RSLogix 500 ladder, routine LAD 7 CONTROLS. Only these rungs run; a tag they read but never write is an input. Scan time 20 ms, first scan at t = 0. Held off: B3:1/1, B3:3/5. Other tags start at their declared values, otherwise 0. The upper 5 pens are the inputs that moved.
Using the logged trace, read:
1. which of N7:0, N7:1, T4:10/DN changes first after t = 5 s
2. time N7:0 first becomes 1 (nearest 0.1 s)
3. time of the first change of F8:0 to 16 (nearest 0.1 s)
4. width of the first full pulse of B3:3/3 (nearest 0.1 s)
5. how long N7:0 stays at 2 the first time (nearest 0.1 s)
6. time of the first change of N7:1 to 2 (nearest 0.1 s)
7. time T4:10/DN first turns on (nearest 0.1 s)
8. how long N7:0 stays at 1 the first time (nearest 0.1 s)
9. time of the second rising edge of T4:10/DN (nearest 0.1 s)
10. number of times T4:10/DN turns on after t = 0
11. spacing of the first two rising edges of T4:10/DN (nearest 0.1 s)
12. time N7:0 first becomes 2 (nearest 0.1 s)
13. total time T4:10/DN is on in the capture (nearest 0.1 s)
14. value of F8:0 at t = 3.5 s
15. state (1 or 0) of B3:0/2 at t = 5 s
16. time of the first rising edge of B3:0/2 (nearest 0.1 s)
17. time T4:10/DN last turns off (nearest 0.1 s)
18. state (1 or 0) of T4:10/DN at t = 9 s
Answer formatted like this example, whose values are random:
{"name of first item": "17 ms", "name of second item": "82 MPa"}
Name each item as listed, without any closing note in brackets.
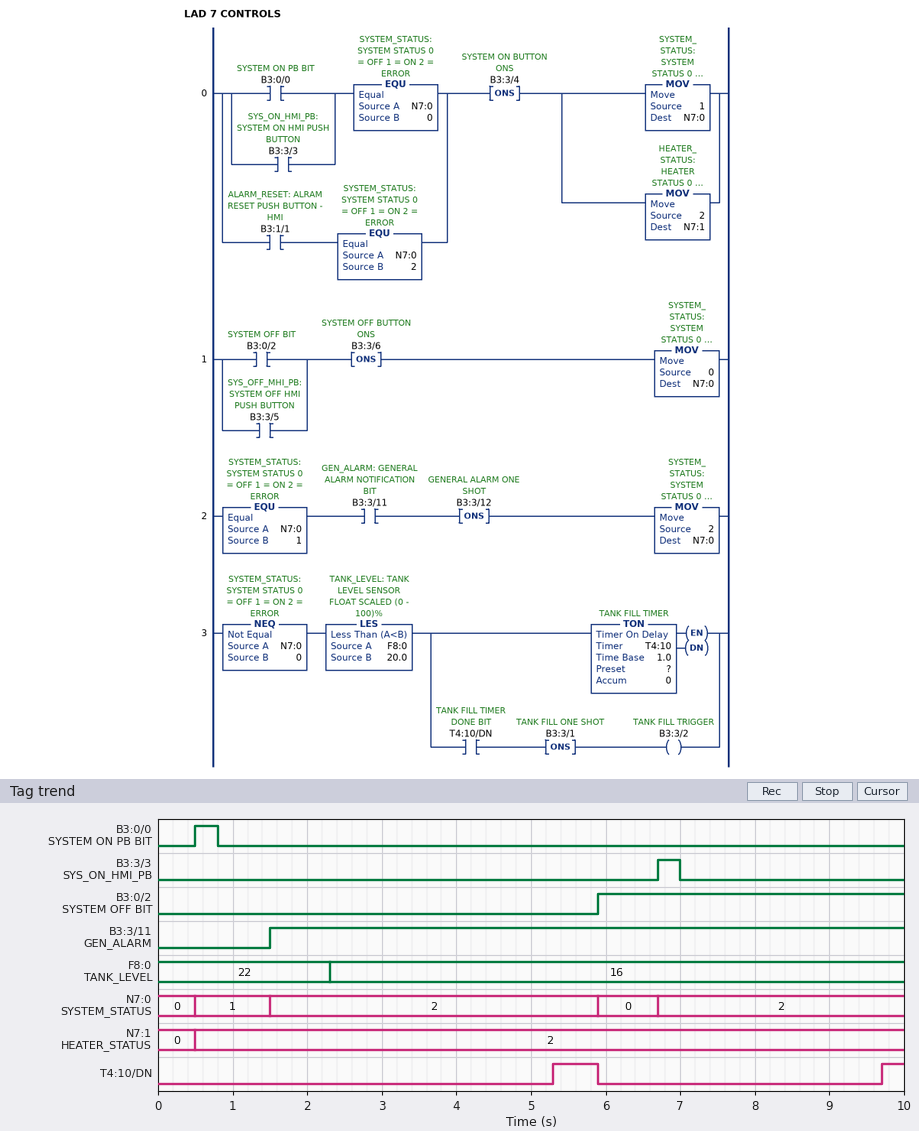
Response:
{"which of N7:0, N7:1, T4:10/DN changes first after t = 5 s": "T4:10/DN", "time N7:0 first becomes 1": "0.5 s", "time of the first change of F8:0 to 16": "2.3 s", "width of the first full pulse of B3:3/3": "0.3 s", "how long N7:0 stays at 2 the first time": "4.4 s", "time of the first change of N7:1 to 2": "0.5 s", "time T4:10/DN first turns on": "5.3 s", "how long N7:0 stays at 1 the first time": "1.0 s", "time of the second rising edge of T4:10/DN": "9.7 s", "number of times T4:10/DN turns on after t = 0": "2", "spacing of the first two rising edges of T4:10/DN": "4.4 s", "time N7:0 first becomes 2": "1.5 s", "total time T4:10/DN is on in the capture": "0.9 s", "value of F8:0 at t = 3.5 s": "16", "state (1 or 0) of B3:0/2 at t = 5 s": "0", "time of the first rising edge of B3:0/2": "5.9 s", "time T4:10/DN last turns off": "5.9 s", "state (1 or 0) of T4:10/DN at t = 9 s": "0"}
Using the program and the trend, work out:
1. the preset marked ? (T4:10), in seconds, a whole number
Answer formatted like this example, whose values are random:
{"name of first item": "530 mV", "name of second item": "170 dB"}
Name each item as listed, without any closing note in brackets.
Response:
{"the preset marked ? (T4:10), in seconds, a whole number": "3 s"}
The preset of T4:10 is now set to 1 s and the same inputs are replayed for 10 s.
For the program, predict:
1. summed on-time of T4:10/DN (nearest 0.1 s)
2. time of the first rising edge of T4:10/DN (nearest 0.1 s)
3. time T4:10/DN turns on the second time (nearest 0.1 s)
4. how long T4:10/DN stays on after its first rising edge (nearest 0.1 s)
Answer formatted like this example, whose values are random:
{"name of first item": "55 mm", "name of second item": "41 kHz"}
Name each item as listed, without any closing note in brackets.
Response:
{"summed on-time of T4:10/DN": "4.9 s", "time of the first rising edge of T4:10/DN": "3.3 s", "time T4:10/DN turns on the second time": "7.7 s", "how long T4:10/DN stays on after its first rising edge": "2.6 s"}
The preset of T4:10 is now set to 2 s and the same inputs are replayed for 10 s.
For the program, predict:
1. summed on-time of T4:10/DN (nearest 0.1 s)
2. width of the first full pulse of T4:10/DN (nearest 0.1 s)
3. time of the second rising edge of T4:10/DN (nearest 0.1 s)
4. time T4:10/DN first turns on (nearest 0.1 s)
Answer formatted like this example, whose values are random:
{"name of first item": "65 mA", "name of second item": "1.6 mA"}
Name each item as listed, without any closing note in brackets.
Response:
{"summed on-time of T4:10/DN": "2.9 s", "width of the first full pulse of T4:10/DN": "1.6 s", "time of the second rising edge of T4:10/DN": "8.7 s", "time T4:10/DN first turns on": "4.3 s"}
